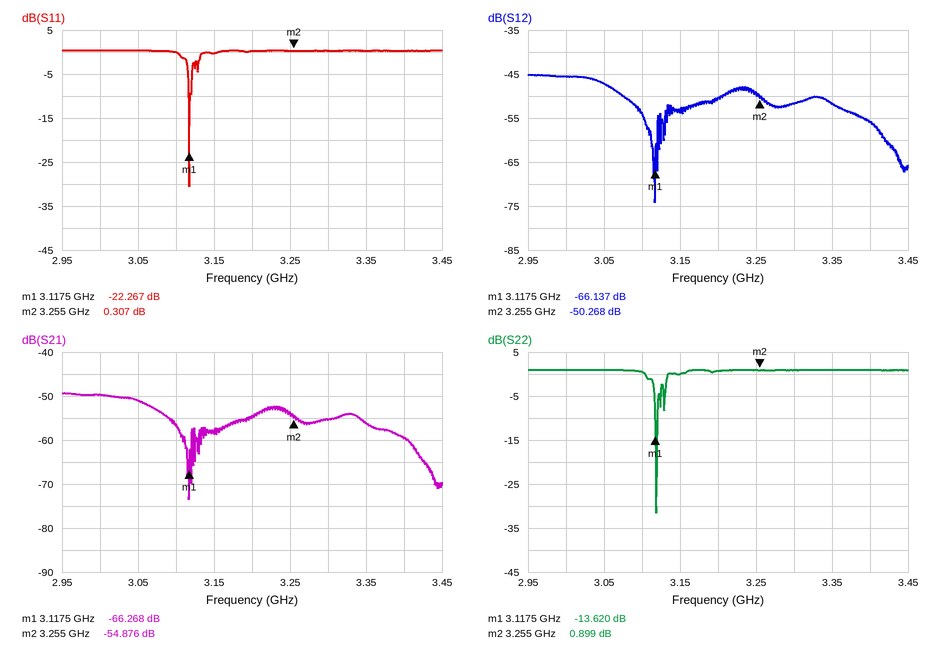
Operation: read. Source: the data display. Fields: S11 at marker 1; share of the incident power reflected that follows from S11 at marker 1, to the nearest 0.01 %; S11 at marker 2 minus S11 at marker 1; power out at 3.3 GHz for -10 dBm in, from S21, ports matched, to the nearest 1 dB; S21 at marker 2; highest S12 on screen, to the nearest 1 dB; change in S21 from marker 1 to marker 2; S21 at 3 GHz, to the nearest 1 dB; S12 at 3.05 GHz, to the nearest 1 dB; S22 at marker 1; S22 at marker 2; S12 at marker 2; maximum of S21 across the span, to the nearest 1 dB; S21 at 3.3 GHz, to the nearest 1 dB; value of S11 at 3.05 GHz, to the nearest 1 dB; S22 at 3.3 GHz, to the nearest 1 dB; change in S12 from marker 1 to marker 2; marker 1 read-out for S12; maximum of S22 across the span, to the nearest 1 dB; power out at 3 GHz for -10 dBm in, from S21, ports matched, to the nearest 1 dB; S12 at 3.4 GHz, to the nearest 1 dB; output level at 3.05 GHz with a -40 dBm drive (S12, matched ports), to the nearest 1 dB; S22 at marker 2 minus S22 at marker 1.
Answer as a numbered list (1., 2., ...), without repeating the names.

1. -22.267 dB
2. 0.59 %
3. 22.574 dB
4. -65 dBm
5. -54.876 dB
6. -45 dB
7. 11.392 dB
8. -50 dB
9. -47 dB
10. -13.620 dB
11. 0.899 dB
12. -50.268 dB
13. -49 dB
14. -55 dB
15. 0 dB
16. 1 dB
17. 15.869 dB
18. -66.137 dB
19. 1 dB
20. -60 dBm
21. -56 dB
22. -87 dBm
23. 14.519 dB
